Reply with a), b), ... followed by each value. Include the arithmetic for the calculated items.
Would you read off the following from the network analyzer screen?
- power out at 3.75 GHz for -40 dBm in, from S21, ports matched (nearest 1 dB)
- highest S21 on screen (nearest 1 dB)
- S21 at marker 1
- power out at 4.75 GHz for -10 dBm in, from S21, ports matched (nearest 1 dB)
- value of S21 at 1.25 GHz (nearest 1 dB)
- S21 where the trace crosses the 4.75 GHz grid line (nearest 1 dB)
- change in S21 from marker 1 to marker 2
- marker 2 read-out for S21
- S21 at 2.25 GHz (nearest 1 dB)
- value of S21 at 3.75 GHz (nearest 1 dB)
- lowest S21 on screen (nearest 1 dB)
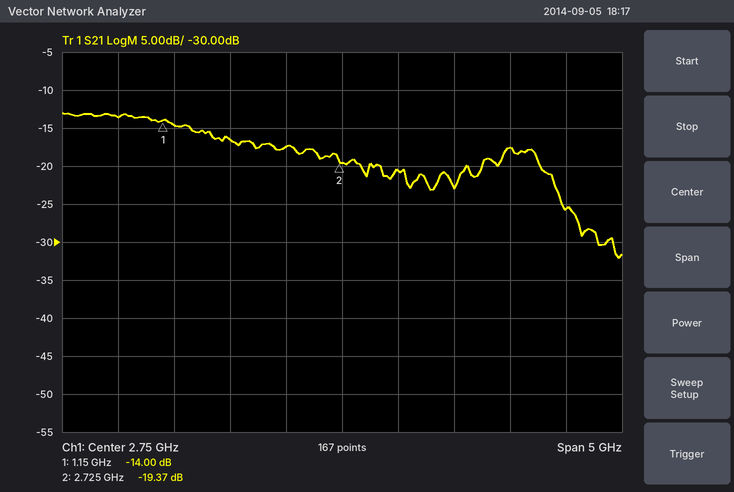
a) -40 dBm + (-23 dB) = -63 dBm
b) -13 dB
c) -14.00 dB
d) -10 dBm + (-26 dB) = -36 dBm
e) -15 dB
f) -26 dB
g) -19.37 − (-14) = -5.37 dB
h) -19.37 dB
i) -17 dB
j) -23 dB
k) -32 dB
